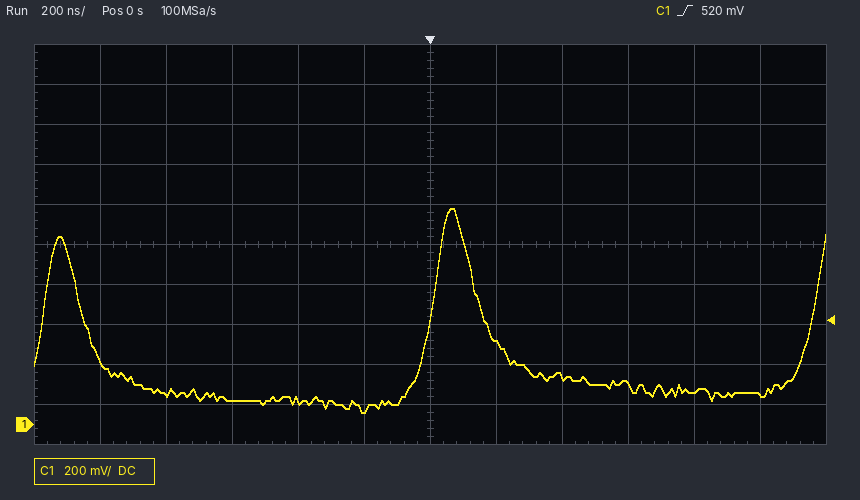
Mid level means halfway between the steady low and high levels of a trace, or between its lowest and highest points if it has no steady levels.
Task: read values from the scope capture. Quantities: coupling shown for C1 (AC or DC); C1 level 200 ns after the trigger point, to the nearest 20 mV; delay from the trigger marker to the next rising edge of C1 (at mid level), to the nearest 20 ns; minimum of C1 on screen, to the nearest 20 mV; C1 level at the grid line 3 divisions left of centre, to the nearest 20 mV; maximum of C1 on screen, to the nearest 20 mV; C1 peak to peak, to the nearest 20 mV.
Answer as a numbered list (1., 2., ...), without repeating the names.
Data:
1. DC
2. 420 mV
3. 1.16 µs
4. 60 mV
5. 120 mV
6. 1.08 V
7. 1.02 V
